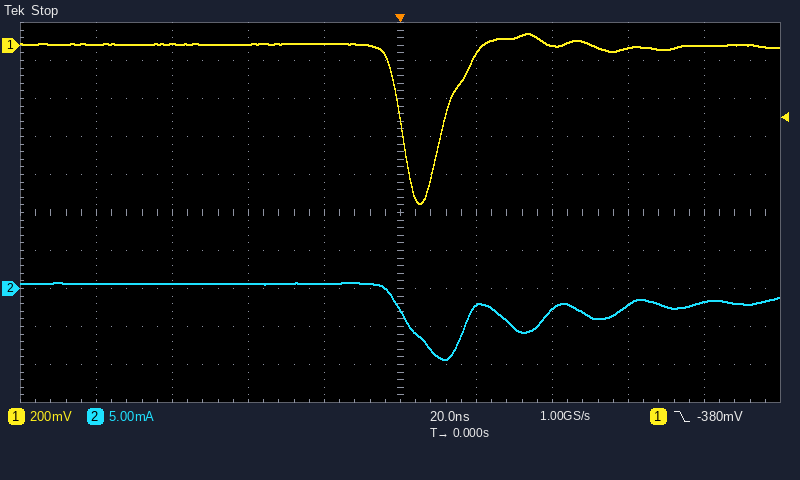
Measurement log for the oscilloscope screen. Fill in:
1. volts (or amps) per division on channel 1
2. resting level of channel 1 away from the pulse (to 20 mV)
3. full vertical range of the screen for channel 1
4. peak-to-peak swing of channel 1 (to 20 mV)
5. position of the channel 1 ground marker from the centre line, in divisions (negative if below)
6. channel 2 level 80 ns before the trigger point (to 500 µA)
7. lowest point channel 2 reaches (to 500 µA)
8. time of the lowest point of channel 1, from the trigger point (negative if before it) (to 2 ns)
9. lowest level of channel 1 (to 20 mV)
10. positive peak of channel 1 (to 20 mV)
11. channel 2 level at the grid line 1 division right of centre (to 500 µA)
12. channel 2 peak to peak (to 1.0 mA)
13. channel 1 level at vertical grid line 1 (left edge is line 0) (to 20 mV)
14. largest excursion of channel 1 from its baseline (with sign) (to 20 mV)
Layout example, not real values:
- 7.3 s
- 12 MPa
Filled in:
- 200 mV
- 0 mV
- 2 V
- 900 mV
- +4.4 div
- 500 µA
- -9.5 mA
- +6 ns
- -840 mV
- 60 mV
- -2.5 mA
- 10.0 mA
- 0 mV
- -840 mV
